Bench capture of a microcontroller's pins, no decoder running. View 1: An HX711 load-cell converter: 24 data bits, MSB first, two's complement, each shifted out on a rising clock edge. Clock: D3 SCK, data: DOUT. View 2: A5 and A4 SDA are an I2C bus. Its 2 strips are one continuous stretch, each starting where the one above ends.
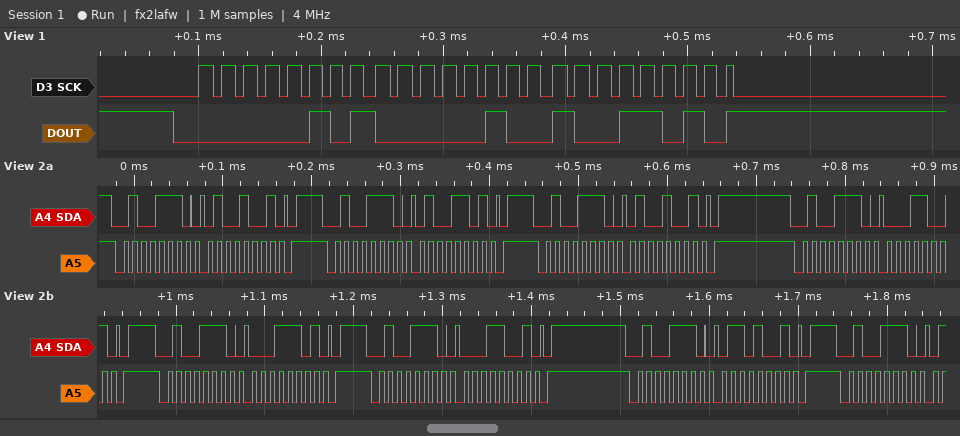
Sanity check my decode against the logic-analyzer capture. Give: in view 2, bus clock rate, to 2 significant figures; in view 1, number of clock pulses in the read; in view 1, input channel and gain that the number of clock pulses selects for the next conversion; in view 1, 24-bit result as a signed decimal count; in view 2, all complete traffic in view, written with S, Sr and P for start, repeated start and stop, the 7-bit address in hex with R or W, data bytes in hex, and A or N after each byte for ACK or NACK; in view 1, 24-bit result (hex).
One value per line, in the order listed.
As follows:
100 kHz
25
channel A, gain 128
328858
S 27W A 49 A P S 27W A 4D A P S 27W A 49 A P S 27W A 19 A P S 27W A 1D A P S 27W A 19 A P S 27W A 69 A P S 27W A
0x05049A
